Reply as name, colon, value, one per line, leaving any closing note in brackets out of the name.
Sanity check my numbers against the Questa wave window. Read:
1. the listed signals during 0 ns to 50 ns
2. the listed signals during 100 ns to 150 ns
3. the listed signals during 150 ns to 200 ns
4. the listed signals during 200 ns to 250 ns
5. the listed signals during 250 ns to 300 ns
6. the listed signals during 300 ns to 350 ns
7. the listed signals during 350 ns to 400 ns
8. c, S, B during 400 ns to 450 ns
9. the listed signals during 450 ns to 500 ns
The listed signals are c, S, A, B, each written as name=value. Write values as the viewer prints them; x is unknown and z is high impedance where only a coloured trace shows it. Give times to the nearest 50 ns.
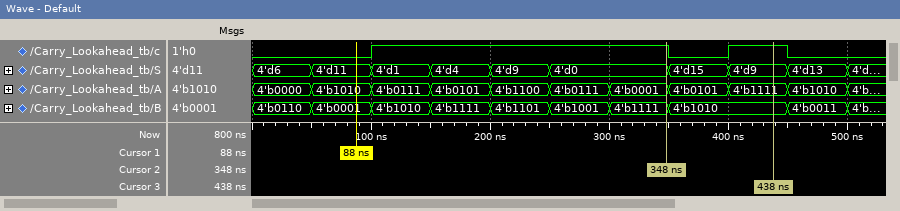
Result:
the listed signals during 0 ns to 50 ns: c=0, S=4'd6, A=4'b0000, B=4'b0110
the listed signals during 100 ns to 150 ns: c=1, S=4'd1, A=4'b0111, B=4'b1010
the listed signals during 150 ns to 200 ns: c=1, S=4'd4, A=4'b0101, B=4'b1111
the listed signals during 200 ns to 250 ns: c=1, S=4'd9, A=4'b1100, B=4'b1101
the listed signals during 250 ns to 300 ns: c=1, S=4'd0, A=4'b0111, B=4'b1001
the listed signals during 300 ns to 350 ns: c=1, S=4'd0, A=4'b0001, B=4'b1111
the listed signals during 350 ns to 400 ns: c=0, S=4'd15, A=4'b0101, B=4'b1010
c, S, B during 400 ns to 450 ns: c=1, S=4'd9, B=4'b1010
the listed signals during 450 ns to 500 ns: c=0, S=4'd13, A=4'b1010, B=4'b0011
